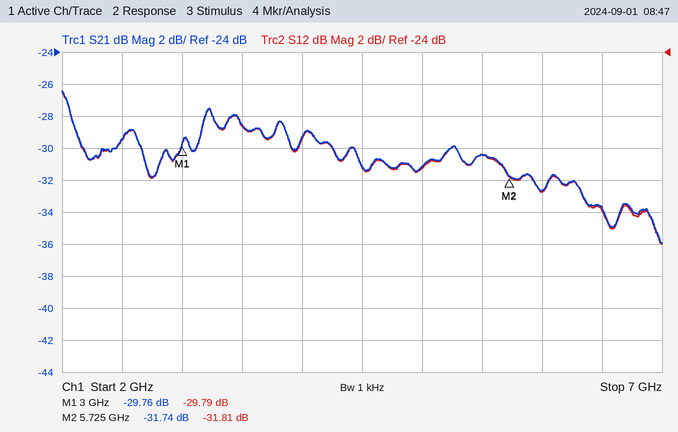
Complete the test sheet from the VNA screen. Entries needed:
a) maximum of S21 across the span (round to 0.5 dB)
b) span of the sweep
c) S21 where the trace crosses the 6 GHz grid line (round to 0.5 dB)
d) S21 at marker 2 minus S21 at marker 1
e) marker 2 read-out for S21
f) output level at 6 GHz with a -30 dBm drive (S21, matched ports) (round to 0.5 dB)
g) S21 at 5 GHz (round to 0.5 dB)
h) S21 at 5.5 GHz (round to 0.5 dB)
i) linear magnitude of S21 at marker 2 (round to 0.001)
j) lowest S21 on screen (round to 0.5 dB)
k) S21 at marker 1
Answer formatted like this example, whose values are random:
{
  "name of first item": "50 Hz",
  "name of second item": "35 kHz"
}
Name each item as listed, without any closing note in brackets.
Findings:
{
  "maximum of S21 across the span": "-26.5 dB",
  "span of the sweep": "5 GHz",
  "S21 where the trace crosses the 6 GHz grid line": "-32.5 dB",
  "S21 at marker 2 minus S21 at marker 1": "-1.98 dB",
  "marker 2 read-out for S21": "-31.74 dB",
  "output level at 6 GHz with a -30 dBm drive (S21, matched ports)": "-62.5 dBm",
  "S21 at 5 GHz": "-31.0 dB",
  "S21 at 5.5 GHz": "-30.5 dB",
  "linear magnitude of S21 at marker 2": "0.026",
  "lowest S21 on screen": "-36.0 dB",
  "S21 at marker 1": "-29.76 dB"
}
